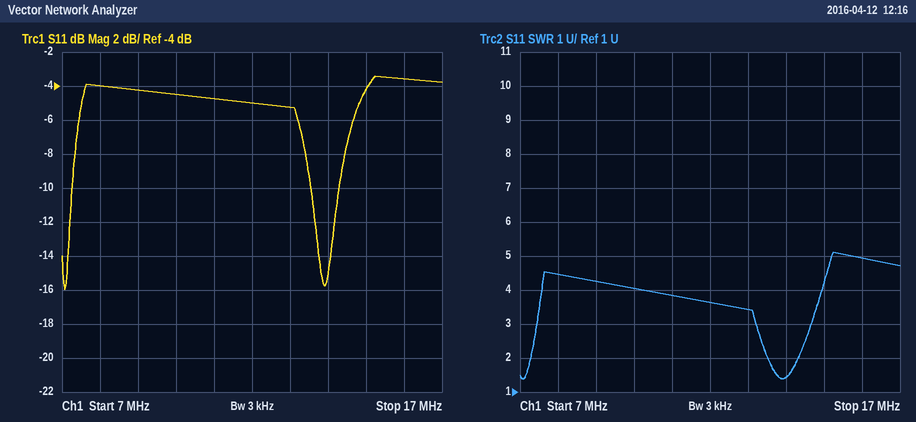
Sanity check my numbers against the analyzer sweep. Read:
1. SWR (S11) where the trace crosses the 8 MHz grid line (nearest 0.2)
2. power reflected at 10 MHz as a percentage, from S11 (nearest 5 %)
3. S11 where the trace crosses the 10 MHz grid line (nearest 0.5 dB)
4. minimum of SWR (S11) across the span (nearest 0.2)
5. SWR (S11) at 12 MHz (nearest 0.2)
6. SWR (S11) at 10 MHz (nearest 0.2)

4.4
35 %
-4.5 dB
1.4
3.6
4.0
